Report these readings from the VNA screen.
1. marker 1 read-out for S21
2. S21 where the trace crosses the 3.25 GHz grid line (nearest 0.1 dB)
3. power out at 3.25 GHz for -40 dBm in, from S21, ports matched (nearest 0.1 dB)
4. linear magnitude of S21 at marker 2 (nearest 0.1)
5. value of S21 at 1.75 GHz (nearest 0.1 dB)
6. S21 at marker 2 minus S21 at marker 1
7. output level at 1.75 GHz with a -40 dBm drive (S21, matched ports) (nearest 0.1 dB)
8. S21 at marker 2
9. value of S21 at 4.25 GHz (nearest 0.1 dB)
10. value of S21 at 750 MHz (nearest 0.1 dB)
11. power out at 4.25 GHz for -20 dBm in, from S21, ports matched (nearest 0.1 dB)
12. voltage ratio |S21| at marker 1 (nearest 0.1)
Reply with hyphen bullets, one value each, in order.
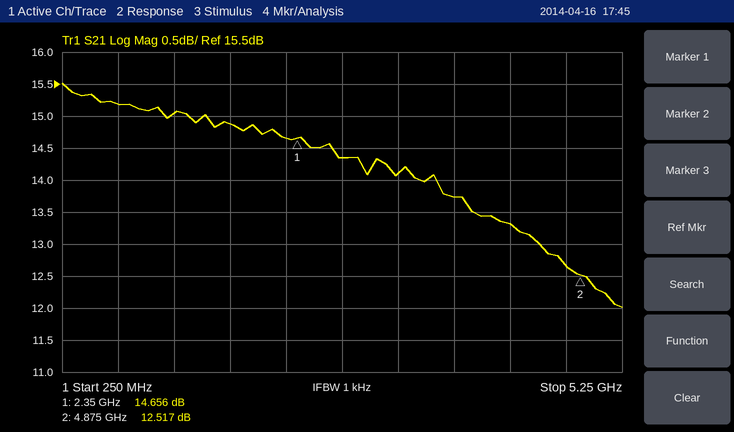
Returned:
- 14.656 dB
- 14.1 dB
- -25.9 dBm
- 4.2
- 14.9 dB
- -2.139 dB
- -25.1 dBm
- 12.517 dB
- 13.3 dB
- 15.2 dB
- -6.7 dBm
- 5.4
